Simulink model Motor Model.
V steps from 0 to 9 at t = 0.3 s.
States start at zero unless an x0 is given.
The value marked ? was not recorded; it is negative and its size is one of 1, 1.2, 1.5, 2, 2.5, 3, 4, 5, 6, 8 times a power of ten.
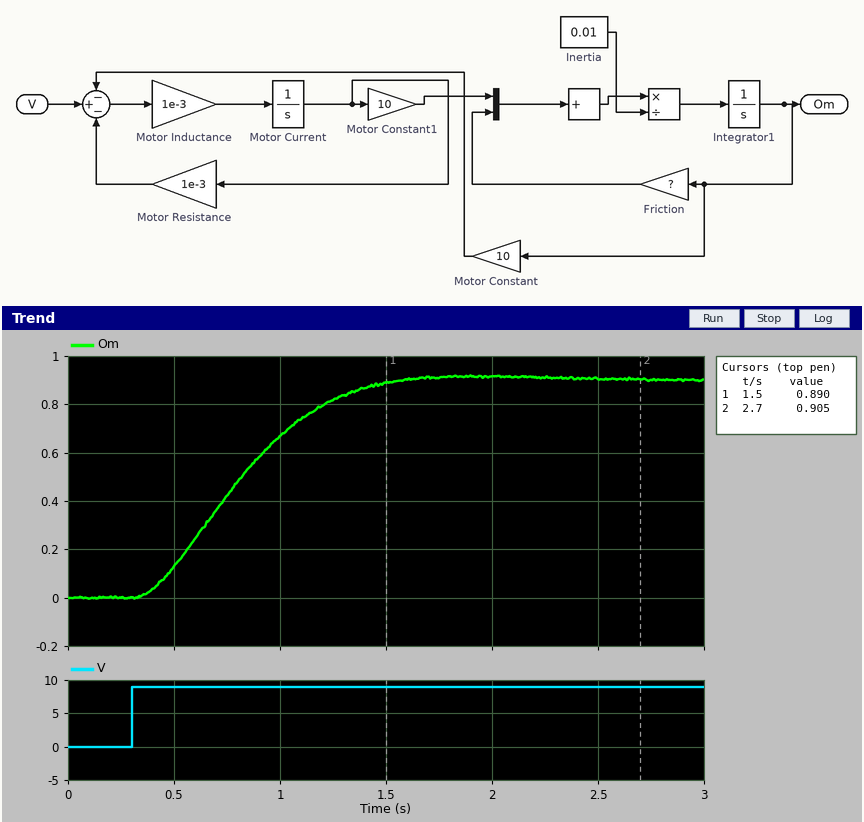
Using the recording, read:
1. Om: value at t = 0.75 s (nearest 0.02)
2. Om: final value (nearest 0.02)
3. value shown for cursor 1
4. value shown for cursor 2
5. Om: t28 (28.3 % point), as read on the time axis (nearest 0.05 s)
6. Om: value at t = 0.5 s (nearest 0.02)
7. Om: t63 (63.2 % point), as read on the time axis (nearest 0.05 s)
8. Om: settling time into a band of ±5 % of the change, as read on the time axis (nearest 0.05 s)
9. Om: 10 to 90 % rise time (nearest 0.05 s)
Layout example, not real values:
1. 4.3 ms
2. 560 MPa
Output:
1. 0.42
2. 0.90
3. 0.890
4. 0.905
5. 0.60 s
6. 0.12
7. 0.90 s
8. 1.35 s
9. 0.75 s
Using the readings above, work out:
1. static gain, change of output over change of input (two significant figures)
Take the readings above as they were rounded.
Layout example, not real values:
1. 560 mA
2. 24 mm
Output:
1. 0.10
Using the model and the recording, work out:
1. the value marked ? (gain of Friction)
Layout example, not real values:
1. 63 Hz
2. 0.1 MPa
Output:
1. -0.05
